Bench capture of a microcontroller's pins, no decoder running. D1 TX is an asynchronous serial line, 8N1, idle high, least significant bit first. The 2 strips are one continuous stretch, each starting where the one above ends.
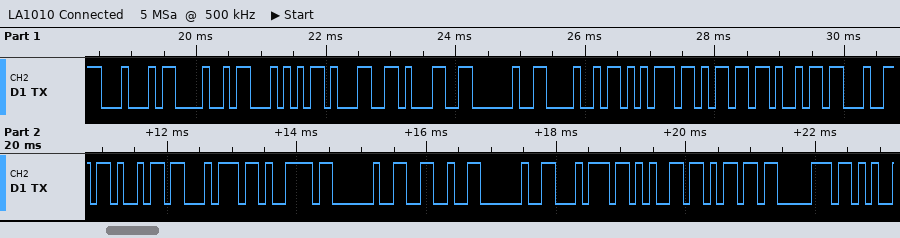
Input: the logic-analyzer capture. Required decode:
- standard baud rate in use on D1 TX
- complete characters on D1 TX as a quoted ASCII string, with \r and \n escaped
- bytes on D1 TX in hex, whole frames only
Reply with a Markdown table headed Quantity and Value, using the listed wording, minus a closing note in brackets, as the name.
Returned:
| Quantity | Value |
|---|---|
| standard baud rate in use on D1 TX | 9600 baud |
| complete characters on D1 TX as a quoted ASCII string, with \r and \n escaped | "DHT11 Humidity & temp" |
| bytes on D1 TX in hex, whole frames only | 44 48 54 31 31 20 48 75 6D 69 64 69 74 79 20 26 20 74 65 6D 70 |
